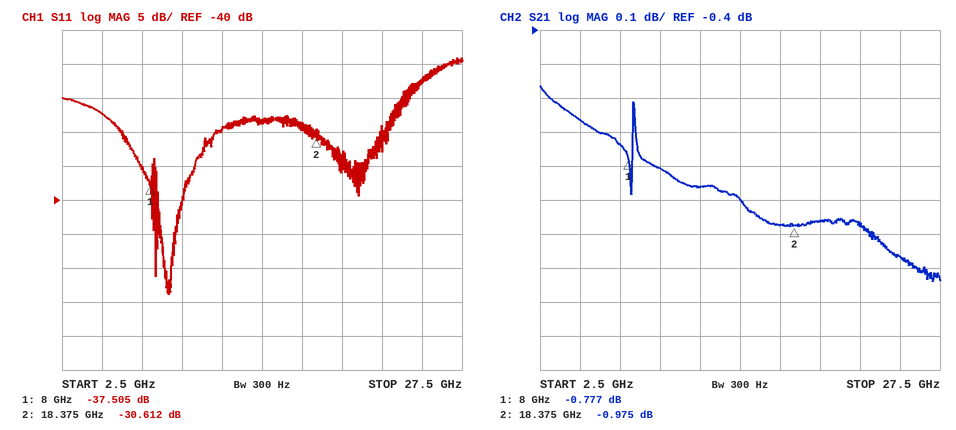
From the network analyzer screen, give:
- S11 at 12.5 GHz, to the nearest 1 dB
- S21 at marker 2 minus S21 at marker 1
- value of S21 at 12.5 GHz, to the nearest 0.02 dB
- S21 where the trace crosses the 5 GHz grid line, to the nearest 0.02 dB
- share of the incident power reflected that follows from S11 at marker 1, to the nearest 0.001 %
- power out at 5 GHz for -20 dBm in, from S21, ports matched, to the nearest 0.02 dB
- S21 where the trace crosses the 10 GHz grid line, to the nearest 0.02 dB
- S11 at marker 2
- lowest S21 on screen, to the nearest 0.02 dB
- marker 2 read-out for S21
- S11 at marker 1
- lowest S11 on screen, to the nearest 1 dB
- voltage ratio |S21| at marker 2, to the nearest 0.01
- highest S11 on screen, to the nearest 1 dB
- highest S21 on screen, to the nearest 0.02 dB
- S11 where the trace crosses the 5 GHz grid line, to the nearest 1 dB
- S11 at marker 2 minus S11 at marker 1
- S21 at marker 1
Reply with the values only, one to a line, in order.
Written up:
-30 dB
-0.198 dB
-0.86 dB
-0.66 dB
0.018 %
-20.66 dBm
-0.80 dB
-30.612 dB
-1.14 dB
-0.975 dB
-37.505 dB
-54 dB
0.89
-19 dB
-0.56 dB
-27 dB
6.893 dB
-0.777 dB
